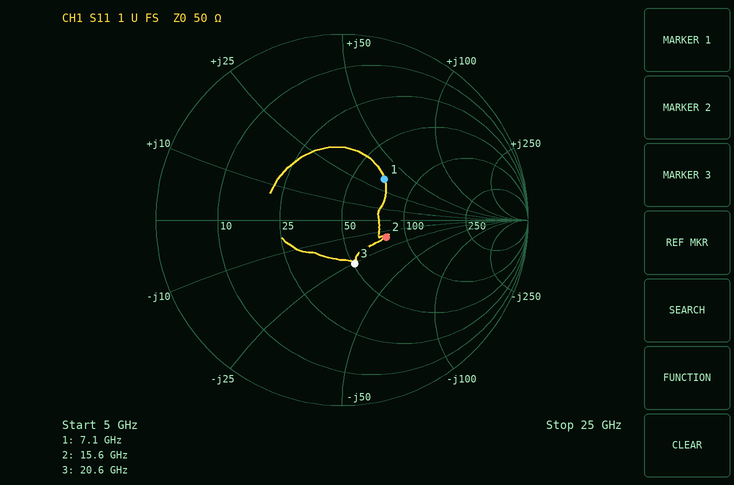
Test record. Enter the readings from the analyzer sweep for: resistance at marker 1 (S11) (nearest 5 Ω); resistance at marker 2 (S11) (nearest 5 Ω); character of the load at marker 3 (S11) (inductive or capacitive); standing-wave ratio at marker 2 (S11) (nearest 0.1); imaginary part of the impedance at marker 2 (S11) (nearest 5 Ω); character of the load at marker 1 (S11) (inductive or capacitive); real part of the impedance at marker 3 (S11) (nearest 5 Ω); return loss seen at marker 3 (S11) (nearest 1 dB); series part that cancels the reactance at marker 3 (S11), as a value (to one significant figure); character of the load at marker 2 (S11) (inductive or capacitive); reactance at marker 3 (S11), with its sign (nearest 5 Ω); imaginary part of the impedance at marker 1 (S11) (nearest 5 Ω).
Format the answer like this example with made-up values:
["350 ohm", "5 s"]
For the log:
["70 Ω", "80 Ω", "capacitive", "1.7", "-15 Ω", "inductive", "50 Ω", "12 dB", "200 pH", "capacitive", "-25 Ω", "+35 Ω"]
